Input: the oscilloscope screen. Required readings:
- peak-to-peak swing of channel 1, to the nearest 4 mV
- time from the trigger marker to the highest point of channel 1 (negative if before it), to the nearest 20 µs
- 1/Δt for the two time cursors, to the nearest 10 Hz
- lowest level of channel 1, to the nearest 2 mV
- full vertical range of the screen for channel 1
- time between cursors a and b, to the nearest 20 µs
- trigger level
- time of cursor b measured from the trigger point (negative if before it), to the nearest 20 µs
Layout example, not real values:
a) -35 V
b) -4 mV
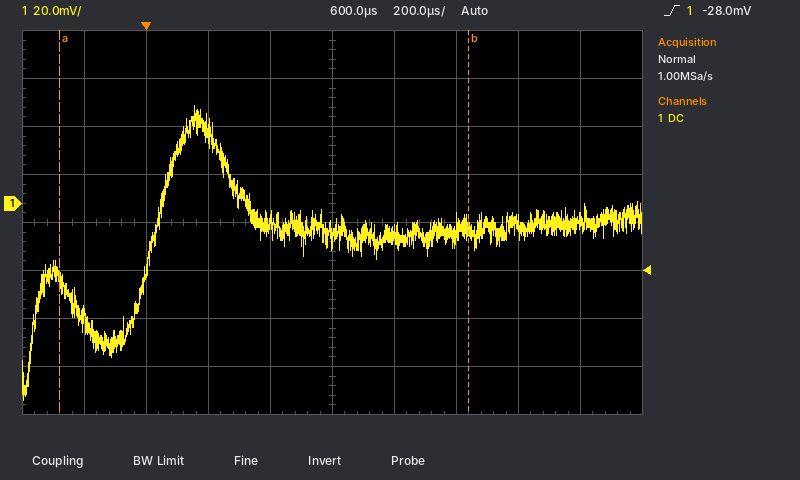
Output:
a) 124 mV
b) +160 µs
c) 760 Hz
d) -82 mV
e) 160 mV
f) 1.32 ms
g) -28.0 mV
h) +1.04 ms
